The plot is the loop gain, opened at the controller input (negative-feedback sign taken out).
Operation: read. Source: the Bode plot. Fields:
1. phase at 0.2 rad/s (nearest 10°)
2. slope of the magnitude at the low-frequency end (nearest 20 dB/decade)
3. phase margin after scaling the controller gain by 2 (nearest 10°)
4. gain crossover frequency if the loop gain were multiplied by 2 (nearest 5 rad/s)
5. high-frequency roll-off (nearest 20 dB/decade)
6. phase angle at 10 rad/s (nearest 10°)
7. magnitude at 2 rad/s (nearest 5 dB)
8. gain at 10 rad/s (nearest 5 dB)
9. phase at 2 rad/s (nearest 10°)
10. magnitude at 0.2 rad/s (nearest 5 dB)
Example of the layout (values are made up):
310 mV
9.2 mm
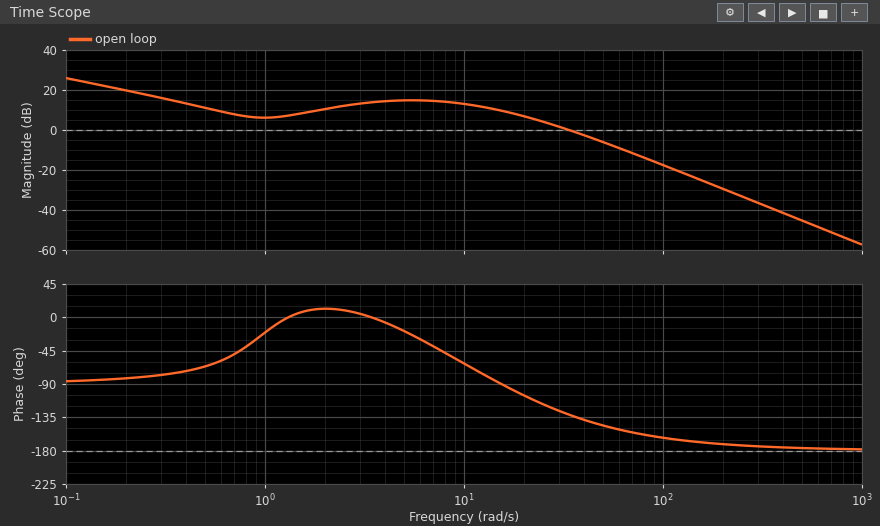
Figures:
-80°
-20 dB/decade
30°
50 rad/s
-40 dB/decade
-60°
10 dB
15 dB
10°
20 dB
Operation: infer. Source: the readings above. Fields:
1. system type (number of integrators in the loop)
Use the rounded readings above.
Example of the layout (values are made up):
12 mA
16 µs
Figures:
1
